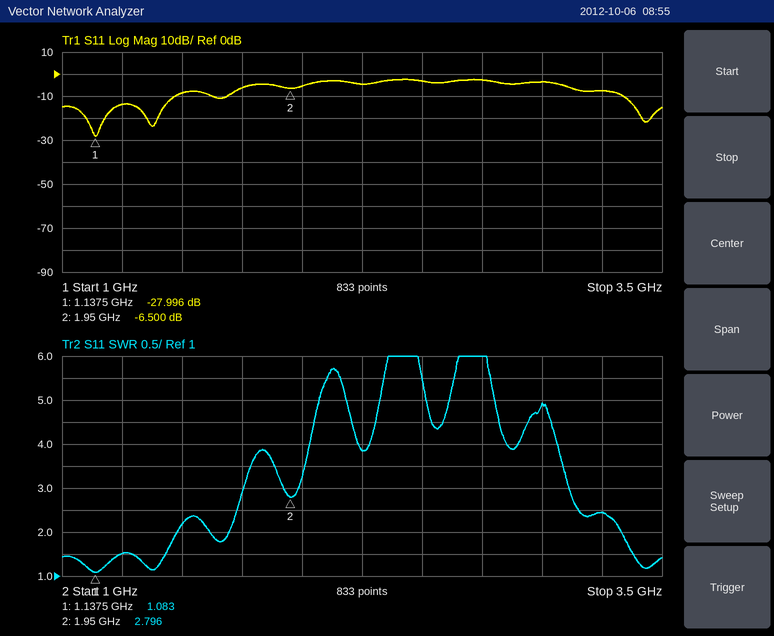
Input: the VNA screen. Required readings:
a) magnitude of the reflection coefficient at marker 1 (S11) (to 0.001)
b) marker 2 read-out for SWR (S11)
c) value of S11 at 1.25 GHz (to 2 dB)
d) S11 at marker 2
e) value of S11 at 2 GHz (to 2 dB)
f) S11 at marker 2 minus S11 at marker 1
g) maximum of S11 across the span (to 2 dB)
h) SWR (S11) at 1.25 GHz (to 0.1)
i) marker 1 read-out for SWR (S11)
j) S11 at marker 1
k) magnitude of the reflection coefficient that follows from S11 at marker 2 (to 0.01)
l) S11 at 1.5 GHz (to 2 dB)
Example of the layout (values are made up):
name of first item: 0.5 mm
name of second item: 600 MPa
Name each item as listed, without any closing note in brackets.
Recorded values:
magnitude of the reflection coefficient at marker 1 (S11): 0.040
marker 2 read-out for SWR: 2.796
value of S11 at 1.25 GHz: -14 dB
S11 at marker 2: -6.500 dB
value of S11 at 2 GHz: -6 dB
S11 at marker 2 minus S11 at marker 1: 21.496 dB
maximum of S11 across the span: -2 dB
SWR (S11) at 1.25 GHz: 1.5
marker 1 read-out for SWR: 1.083
S11 at marker 1: -27.996 dB
magnitude of the reflection coefficient that follows from S11 at marker 2: 0.47
S11 at 1.5 GHz: -8 dB
